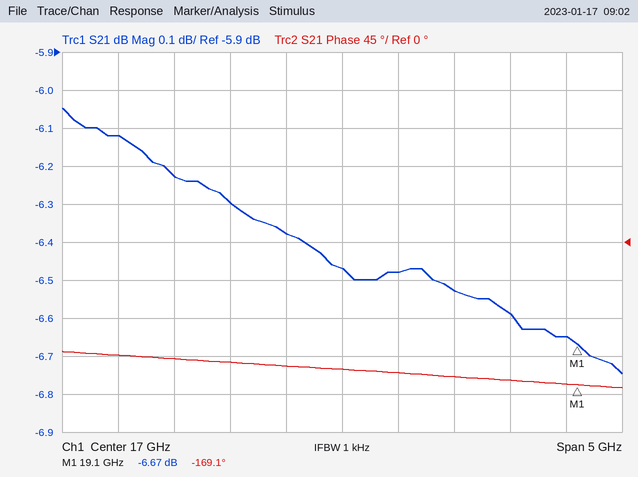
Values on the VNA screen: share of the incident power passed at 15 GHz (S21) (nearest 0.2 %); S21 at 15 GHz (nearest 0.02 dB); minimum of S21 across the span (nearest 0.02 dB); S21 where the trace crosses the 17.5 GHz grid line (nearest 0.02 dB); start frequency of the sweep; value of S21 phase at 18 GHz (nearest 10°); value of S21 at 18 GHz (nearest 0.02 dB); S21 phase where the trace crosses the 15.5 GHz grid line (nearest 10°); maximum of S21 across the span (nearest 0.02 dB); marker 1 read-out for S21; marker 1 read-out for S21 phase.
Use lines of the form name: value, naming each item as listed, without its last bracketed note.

share of the incident power passed at 15 GHz (S21): 24.4 %
S21 at 15 GHz: -6.12 dB
minimum of S21 across the span: -6.74 dB
S21 where the trace crosses the 17.5 GHz grid line: -6.48 dB
start frequency of the sweep: 14.5 GHz
value of S21 phase at 18 GHz: -160°
value of S21 at 18 GHz: -6.52 dB
S21 phase where the trace crosses the 15.5 GHz grid line: -140°
maximum of S21 across the span: -6.04 dB
marker 1 read-out for S21: -6.67 dB
marker 1 read-out for S21 phase: -169.1°
